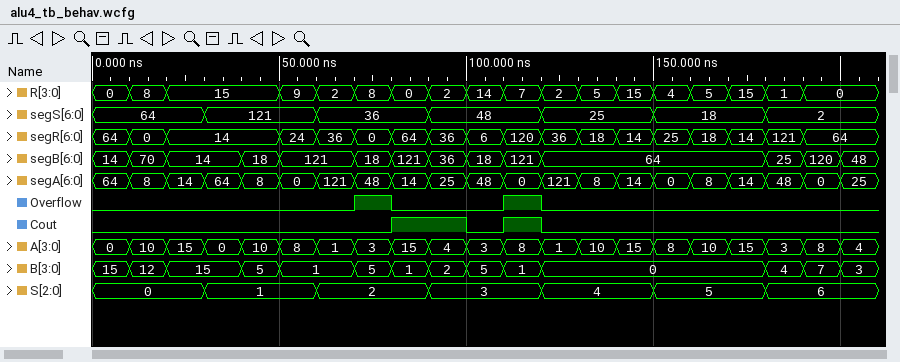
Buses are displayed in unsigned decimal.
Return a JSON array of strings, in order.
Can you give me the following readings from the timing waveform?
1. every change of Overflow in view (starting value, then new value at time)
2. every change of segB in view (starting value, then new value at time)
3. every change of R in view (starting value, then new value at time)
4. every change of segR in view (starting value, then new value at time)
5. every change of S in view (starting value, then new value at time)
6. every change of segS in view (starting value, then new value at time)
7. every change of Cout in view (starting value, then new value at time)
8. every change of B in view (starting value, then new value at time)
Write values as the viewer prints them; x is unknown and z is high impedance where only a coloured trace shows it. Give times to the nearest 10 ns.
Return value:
["0, 1 at 70 ns, 0 at 80 ns, 1 at 110 ns, 0 at 120 ns", "14, 70 at 10 ns, 14 at 20 ns, 18 at 40 ns, 121 at 50 ns, 18 at 70 ns, 121 at 80 ns, 36 at 90 ns, 18 at 100 ns, 121 at 110 ns, 64 at 120 ns, 25 at 180 ns, 120 at 190 ns, 48 at 200 ns", "0, 8 at 10 ns, 15 at 20 ns, 9 at 50 ns, 2 at 60 ns, 8 at 70 ns, 0 at 80 ns, 2 at 90 ns, 14 at 100 ns, 7 at 110 ns, 2 at 120 ns, 5 at 130 ns, 15 at 140 ns, 4 at 150 ns, 5 at 160 ns, 15 at 170 ns, 1 at 180 ns, 0 at 190 ns", "64, 0 at 10 ns, 14 at 20 ns, 24 at 50 ns, 36 at 60 ns, 0 at 70 ns, 64 at 80 ns, 36 at 90 ns, 6 at 100 ns, 120 at 110 ns, 36 at 120 ns, 18 at 130 ns, 14 at 140 ns, 25 at 150 ns, 18 at 160 ns, 14 at 170 ns, 121 at 180 ns, 64 at 190 ns", "0, 1 at 30 ns, 2 at 60 ns, 3 at 90 ns, 4 at 120 ns, 5 at 150 ns, 6 at 180 ns", "64, 121 at 30 ns, 36 at 60 ns, 48 at 90 ns, 25 at 120 ns, 18 at 150 ns, 2 at 180 ns", "0, 1 at 80 ns, 0 at 100 ns, 1 at 110 ns, 0 at 120 ns", "15, 12 at 10 ns, 15 at 20 ns, 5 at 40 ns, 1 at 50 ns, 5 at 70 ns, 1 at 80 ns, 2 at 90 ns, 5 at 100 ns, 1 at 110 ns, 0 at 120 ns, 4 at 180 ns, 7 at 190 ns, 3 at 200 ns"]
